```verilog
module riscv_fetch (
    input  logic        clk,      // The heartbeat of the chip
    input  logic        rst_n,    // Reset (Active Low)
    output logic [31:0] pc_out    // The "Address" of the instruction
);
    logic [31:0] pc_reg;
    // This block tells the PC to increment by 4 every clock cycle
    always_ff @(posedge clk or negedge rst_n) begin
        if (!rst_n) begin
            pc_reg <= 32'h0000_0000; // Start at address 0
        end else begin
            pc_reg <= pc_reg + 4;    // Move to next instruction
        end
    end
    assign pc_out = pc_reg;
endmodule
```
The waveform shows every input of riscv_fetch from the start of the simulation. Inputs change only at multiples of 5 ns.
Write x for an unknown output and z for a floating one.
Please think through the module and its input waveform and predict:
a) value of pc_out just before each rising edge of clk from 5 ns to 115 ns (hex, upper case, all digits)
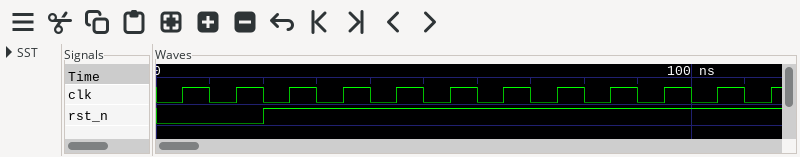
00000000, 00000000, 00000000, 00000004, 00000008, 0000000C, 00000010, 00000014, 00000018, 0000001C, 00000020, 00000024
